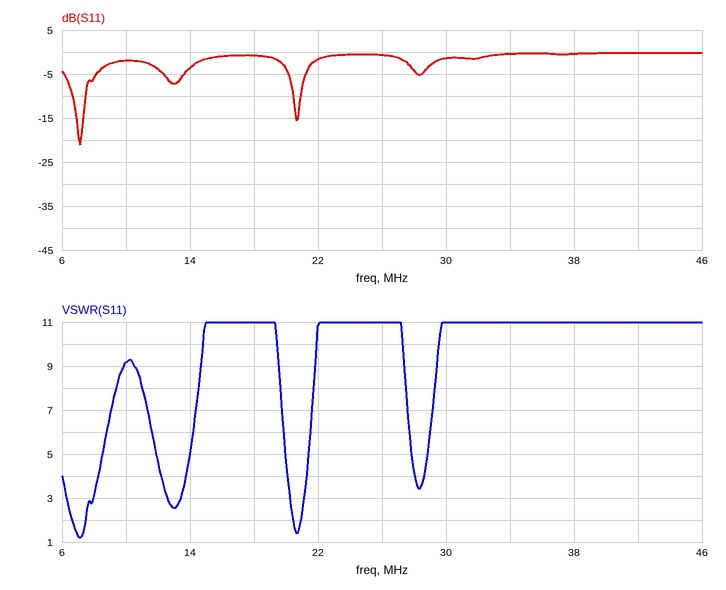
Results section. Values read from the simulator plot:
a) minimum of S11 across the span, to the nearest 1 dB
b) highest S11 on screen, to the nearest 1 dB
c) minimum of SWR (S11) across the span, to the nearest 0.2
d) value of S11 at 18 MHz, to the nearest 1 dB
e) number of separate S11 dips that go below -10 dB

-21 dB
0 dB
1.2
-1 dB
2
